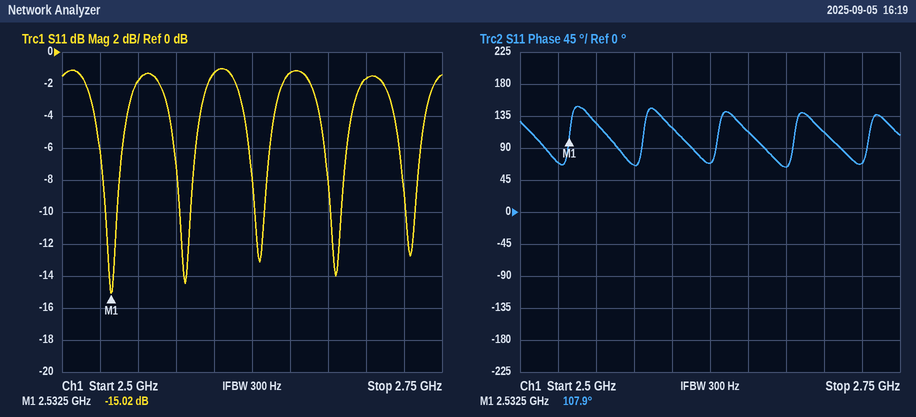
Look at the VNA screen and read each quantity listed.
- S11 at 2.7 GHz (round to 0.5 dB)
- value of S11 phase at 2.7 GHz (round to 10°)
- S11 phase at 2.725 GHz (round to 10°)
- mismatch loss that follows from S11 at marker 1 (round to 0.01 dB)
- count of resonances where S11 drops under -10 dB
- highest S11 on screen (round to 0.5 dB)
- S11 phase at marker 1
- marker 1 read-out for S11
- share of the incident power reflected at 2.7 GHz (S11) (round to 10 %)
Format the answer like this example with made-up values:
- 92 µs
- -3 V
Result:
- -1.5 dB
- 110°
- 70°
- 0.14 dB
- 5
- -1.0 dB
- 107.9°
- -15.02 dB
- 70 %
